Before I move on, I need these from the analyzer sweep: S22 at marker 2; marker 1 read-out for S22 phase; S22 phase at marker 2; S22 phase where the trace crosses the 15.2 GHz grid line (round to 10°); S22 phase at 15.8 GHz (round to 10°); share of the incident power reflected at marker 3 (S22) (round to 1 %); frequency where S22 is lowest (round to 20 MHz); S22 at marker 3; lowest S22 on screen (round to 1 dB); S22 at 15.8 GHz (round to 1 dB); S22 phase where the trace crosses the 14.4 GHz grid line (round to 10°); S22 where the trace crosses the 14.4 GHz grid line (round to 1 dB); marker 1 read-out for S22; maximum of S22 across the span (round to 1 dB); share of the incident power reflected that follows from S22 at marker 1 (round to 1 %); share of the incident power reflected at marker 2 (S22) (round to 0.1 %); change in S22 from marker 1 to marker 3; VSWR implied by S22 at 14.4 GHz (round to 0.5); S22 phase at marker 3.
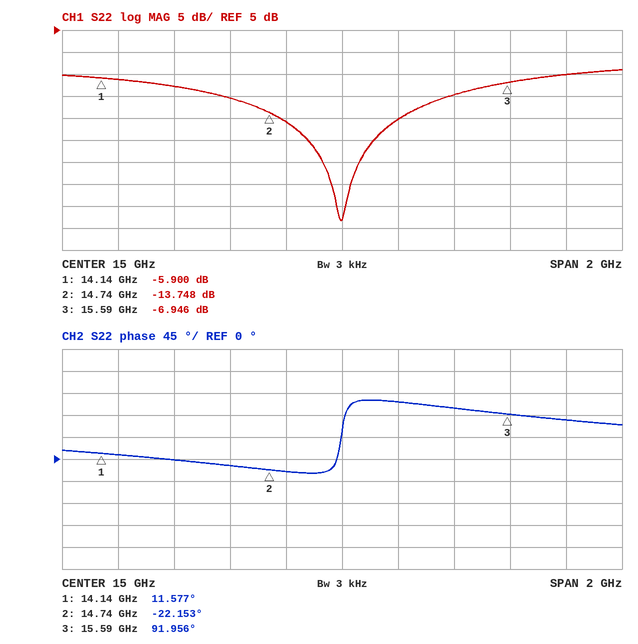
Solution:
-13.748 dB
11.577°
-22.153°
120°
80°
20 %
15.00 GHz
-6.946 dB
-38 dB
-5 dB
0°
-8 dB
-5.900 dB
-4 dB
26 %
4.2 %
-1.046 dB
2.5
91.956°
